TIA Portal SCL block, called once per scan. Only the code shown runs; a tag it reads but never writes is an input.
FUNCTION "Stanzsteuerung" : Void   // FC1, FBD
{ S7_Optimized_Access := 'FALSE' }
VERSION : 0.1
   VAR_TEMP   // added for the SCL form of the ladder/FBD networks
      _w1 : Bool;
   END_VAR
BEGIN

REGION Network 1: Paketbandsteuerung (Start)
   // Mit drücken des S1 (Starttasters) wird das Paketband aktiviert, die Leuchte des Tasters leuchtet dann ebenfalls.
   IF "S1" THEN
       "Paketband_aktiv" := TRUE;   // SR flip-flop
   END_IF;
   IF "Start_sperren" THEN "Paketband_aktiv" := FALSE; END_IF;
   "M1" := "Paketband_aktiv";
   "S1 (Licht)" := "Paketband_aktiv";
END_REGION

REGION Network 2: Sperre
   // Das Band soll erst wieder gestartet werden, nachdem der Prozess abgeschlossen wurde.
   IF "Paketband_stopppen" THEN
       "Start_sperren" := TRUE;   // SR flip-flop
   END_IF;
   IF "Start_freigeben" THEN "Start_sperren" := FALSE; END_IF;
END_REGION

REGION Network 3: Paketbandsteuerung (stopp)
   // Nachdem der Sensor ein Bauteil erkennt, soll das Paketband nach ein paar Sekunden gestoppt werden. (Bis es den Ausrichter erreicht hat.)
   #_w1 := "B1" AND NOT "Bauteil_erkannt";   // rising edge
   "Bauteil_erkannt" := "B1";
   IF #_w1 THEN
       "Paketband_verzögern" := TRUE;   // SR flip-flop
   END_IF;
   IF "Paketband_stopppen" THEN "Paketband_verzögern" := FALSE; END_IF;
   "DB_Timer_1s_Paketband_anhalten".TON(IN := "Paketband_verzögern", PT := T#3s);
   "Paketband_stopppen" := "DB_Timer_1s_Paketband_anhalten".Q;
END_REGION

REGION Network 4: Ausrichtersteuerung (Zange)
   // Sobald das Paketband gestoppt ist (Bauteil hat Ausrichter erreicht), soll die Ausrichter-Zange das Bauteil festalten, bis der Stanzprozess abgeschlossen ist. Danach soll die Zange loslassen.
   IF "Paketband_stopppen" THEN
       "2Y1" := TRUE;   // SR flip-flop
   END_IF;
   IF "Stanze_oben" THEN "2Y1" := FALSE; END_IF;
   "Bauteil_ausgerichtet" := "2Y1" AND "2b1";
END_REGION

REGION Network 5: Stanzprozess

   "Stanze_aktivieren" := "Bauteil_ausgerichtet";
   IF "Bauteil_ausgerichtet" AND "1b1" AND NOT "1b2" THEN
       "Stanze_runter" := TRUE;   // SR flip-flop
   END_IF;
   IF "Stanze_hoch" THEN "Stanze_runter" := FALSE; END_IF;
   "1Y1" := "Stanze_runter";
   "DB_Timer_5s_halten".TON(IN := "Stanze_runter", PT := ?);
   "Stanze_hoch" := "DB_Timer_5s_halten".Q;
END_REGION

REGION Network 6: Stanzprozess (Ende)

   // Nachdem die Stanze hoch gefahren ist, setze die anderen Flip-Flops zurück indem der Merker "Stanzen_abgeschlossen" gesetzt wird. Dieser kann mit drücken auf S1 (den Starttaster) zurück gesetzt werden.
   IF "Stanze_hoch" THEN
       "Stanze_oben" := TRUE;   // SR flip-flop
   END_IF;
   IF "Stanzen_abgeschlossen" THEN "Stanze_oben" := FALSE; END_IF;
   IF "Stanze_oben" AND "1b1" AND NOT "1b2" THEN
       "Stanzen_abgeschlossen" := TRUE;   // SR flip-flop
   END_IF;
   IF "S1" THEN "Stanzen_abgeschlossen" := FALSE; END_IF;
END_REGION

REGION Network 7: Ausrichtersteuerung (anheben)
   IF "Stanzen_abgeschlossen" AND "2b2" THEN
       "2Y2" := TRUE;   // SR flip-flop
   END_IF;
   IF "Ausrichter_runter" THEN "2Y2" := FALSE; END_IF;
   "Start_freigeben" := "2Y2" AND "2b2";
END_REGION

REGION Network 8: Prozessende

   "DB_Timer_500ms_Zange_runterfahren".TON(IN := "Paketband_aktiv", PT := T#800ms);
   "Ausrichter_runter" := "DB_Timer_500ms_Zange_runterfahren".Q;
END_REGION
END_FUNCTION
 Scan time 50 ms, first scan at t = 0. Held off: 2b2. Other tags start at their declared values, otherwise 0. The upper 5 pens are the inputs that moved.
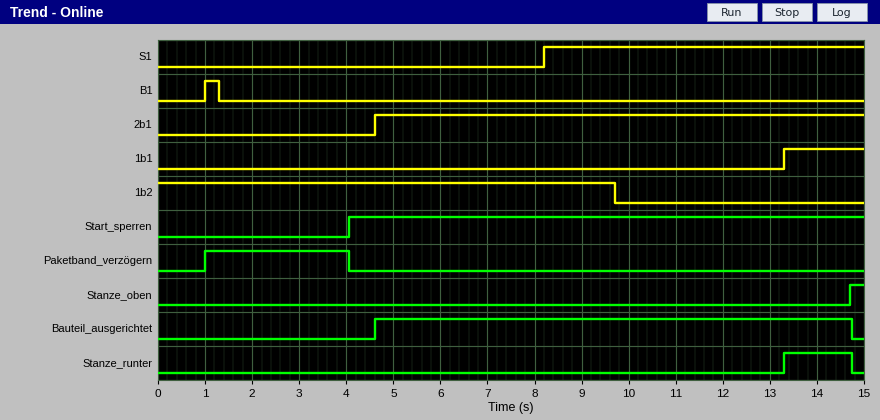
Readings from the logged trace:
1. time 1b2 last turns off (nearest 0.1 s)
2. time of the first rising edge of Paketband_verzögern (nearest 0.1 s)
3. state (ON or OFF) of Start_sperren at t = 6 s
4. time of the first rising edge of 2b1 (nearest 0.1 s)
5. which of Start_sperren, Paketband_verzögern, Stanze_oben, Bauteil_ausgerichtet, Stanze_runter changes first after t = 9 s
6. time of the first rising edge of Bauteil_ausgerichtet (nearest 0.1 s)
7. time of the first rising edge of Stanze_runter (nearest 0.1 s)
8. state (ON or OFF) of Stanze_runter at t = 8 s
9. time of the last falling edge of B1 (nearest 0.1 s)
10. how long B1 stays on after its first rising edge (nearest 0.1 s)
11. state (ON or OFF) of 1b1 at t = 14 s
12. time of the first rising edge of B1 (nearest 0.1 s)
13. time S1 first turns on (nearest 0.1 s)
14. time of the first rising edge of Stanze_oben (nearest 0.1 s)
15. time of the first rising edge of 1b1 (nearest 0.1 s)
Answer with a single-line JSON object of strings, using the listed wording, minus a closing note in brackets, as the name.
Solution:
{"time 1b2 last turns off": "9.7 s", "time of the first rising edge of Paketband_verzögern": "1.0 s", "state (ON or OFF) of Start_sperren at t = 6 s": "ON", "time of the first rising edge of 2b1": "4.6 s", "which of Start_sperren, Paketband_verzögern, Stanze_oben, Bauteil_ausgerichtet, Stanze_runter changes first after t = 9 s": "Stanze_runter", "time of the first rising edge of Bauteil_ausgerichtet": "4.6 s", "time of the first rising edge of Stanze_runter": "13.3 s", "state (ON or OFF) of Stanze_runter at t = 8 s": "OFF", "time of the last falling edge of B1": "1.3 s", "how long B1 stays on after its first rising edge": "0.3 s", "state (ON or OFF) of 1b1 at t = 14 s": "ON", "time of the first rising edge of B1": "1.0 s", "time S1 first turns on": "8.2 s", "time of the first rising edge of Stanze_oben": "14.7 s", "time of the first rising edge of 1b1": "13.3 s"}
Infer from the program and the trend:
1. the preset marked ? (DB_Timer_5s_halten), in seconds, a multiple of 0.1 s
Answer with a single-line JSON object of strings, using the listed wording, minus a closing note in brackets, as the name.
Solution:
{"the preset marked ? (DB_Timer_5s_halten), in seconds, a multiple of 0.1 s": "1.4 s"}
